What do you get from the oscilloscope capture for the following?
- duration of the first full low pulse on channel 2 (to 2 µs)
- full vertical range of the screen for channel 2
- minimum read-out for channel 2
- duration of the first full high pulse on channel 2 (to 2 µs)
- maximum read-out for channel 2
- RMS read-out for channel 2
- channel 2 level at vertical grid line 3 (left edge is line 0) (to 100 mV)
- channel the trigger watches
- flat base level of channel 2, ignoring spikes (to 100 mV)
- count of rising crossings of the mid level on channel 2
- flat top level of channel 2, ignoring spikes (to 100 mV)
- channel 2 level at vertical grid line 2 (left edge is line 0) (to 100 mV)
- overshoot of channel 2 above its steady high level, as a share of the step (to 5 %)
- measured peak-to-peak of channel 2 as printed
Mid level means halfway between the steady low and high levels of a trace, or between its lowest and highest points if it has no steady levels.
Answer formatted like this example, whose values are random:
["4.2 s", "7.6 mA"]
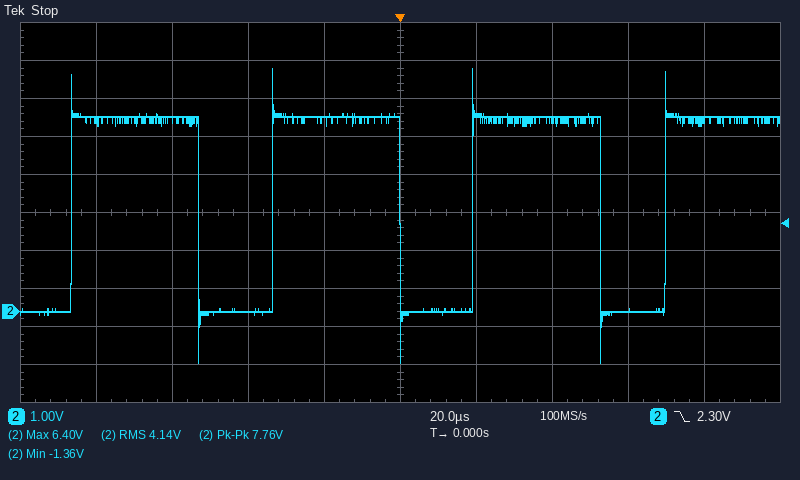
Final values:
["20 µs", "10 V", "-1.36 V", "34 µs", "6.40 V", "4.14 V", "0.0 V", "channel 2", "0.0 V", "4", "5.1 V", "5.0 V", "25 %", "7.76 V"]
